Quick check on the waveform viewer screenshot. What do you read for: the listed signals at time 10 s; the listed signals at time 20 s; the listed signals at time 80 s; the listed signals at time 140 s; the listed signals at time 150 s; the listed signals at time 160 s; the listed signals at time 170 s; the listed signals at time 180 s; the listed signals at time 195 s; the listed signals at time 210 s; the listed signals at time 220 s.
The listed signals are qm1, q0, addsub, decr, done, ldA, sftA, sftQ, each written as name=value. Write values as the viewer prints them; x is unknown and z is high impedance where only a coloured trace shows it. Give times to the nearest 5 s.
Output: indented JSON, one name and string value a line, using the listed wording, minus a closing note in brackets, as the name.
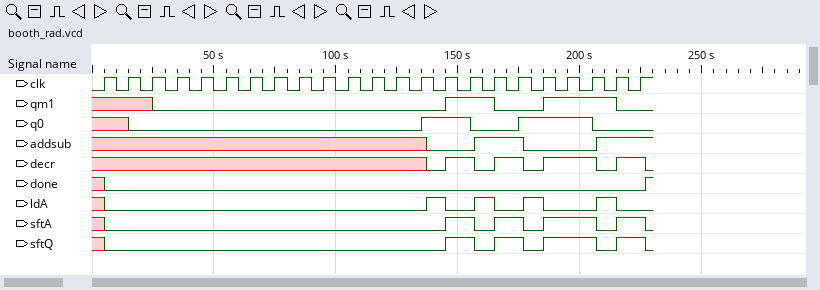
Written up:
{
  "the listed signals at time 10 s": "qm1=x, q0=x, addsub=x, decr=x, done=0, ldA=0, sftA=0, sftQ=0",
  "the listed signals at time 20 s": "qm1=x, q0=0, addsub=x, decr=x, done=0, ldA=0, sftA=0, sftQ=0",
  "the listed signals at time 80 s": "qm1=0, q0=0, addsub=x, decr=x, done=0, ldA=0, sftA=0, sftQ=0",
  "the listed signals at time 140 s": "qm1=0, q0=1, addsub=0, decr=0, done=0, ldA=1, sftA=0, sftQ=0",
  "the listed signals at time 150 s": "qm1=1, q0=1, addsub=0, decr=1, done=0, ldA=0, sftA=1, sftQ=1",
  "the listed signals at time 160 s": "qm1=1, q0=0, addsub=1, decr=0, done=0, ldA=1, sftA=0, sftQ=0",
  "the listed signals at time 170 s": "qm1=0, q0=0, addsub=1, decr=1, done=0, ldA=0, sftA=1, sftQ=1",
  "the listed signals at time 180 s": "qm1=0, q0=1, addsub=0, decr=0, done=0, ldA=1, sftA=0, sftQ=0",
  "the listed signals at time 195 s": "qm1=1, q0=1, addsub=0, decr=1, done=0, ldA=0, sftA=1, sftQ=1",
  "the listed signals at time 210 s": "qm1=1, q0=0, addsub=1, decr=0, done=0, ldA=1, sftA=0, sftQ=0",
  "the listed signals at time 220 s": "qm1=0, q0=0, addsub=1, decr=1, done=0, ldA=0, sftA=1, sftQ=1"
}
